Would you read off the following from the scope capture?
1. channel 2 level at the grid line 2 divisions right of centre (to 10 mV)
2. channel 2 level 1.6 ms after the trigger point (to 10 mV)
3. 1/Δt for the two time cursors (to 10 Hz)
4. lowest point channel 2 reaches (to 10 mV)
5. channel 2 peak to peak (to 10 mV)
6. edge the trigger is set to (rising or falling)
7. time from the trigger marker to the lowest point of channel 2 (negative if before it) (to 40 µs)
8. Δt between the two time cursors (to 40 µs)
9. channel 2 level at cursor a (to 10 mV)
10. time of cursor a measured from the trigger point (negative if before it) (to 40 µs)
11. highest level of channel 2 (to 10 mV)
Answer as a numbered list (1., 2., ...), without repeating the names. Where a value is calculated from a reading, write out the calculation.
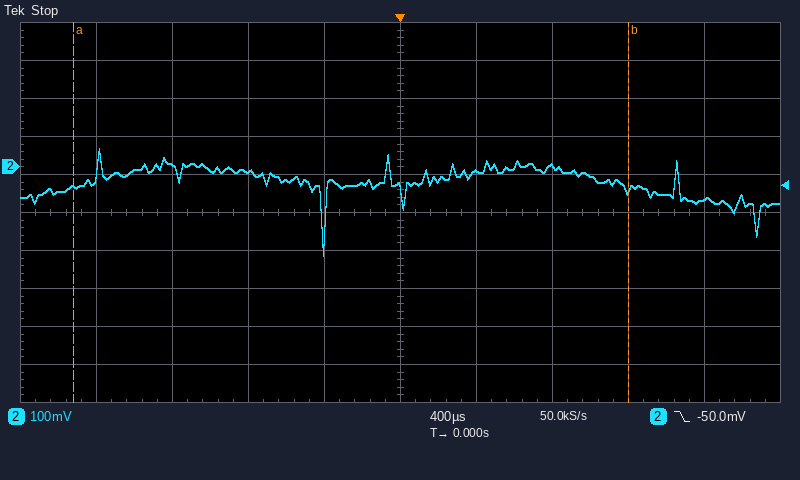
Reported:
1. 0 mV
2. -80 mV
3. 1 / 2.92 ms ≈ 340 Hz
4. -230 mV
5. 50 mV − (-230 mV) = 280 mV
6. falling
7. -400 µs
8. 2.92 ms
9. -50 mV
10. -1.72 ms
11. 50 mV
